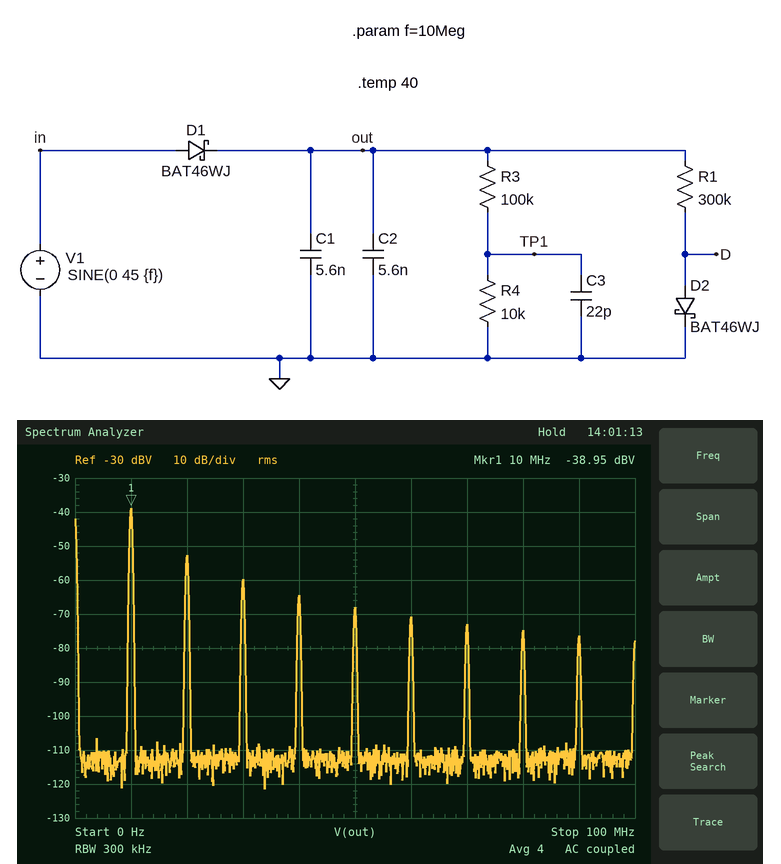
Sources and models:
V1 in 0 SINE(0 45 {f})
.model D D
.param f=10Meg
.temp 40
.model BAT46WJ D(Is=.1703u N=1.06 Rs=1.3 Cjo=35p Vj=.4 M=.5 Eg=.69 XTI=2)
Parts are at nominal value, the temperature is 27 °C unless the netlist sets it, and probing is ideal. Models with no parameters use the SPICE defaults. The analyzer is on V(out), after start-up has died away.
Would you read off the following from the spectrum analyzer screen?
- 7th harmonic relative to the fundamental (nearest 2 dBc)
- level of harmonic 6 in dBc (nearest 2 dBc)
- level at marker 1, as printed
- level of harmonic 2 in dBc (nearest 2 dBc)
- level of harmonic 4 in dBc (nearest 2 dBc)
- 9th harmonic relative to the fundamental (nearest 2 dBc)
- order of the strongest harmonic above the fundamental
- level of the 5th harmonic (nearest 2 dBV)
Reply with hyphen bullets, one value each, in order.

- -34 dBc
- -32 dBc
- -38.95 dBV
- -14 dBc
- -26 dBc
- -38 dBc
- 2
- -68 dBV
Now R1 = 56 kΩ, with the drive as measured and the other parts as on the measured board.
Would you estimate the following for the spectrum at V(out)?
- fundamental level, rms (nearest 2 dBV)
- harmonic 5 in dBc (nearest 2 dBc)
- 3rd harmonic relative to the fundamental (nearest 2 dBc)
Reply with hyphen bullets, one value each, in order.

- -38 dBV
- -26 dBc
- -20 dBc
